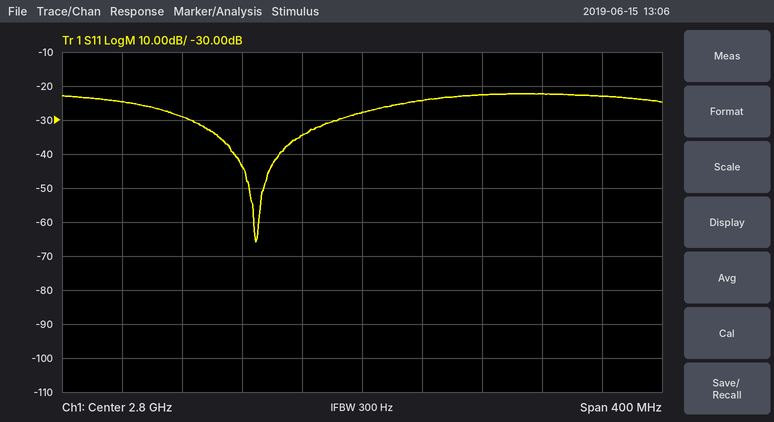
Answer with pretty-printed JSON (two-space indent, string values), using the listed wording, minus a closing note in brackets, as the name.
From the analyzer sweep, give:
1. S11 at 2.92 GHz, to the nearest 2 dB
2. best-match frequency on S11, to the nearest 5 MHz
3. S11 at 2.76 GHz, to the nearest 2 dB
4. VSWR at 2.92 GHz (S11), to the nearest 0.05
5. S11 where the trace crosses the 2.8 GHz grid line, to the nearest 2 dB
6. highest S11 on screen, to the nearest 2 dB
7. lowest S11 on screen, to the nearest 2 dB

{
  "S11 at 2.92 GHz, to the nearest 2 dB": "-22 dB",
  "best-match frequency on S11, to the nearest 5 MHz": "2.730 GHz",
  "S11 at 2.76 GHz, to the nearest 2 dB": "-34 dB",
  "VSWR at 2.92 GHz (S11), to the nearest 0.05": "1.15",
  "S11 where the trace crosses the 2.8 GHz grid line, to the nearest 2 dB": "-28 dB",
  "highest S11 on screen, to the nearest 2 dB": "-22 dB",
  "lowest S11 on screen, to the nearest 2 dB": "-66 dB"
}
